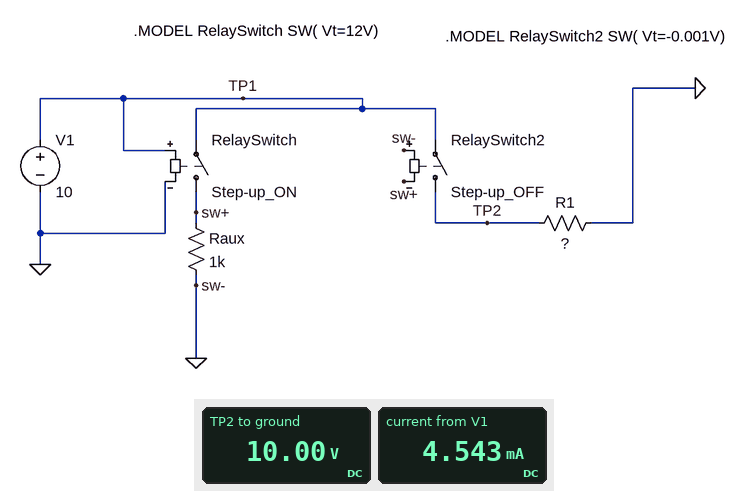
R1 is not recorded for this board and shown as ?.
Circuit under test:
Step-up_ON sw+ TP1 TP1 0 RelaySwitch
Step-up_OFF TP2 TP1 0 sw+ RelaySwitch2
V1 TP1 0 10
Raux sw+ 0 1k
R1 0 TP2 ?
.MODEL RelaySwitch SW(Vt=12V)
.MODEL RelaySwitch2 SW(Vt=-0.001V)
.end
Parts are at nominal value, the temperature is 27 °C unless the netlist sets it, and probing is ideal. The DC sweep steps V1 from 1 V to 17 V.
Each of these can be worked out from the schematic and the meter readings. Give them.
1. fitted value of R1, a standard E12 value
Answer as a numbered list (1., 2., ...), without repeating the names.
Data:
1. 2.2 kΩ
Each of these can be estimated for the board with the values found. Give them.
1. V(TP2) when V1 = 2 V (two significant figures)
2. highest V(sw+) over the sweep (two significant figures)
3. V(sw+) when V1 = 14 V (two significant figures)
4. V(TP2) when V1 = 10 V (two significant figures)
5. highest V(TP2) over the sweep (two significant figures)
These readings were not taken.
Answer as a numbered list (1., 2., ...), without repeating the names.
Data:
1. 2.0 V
2. 17 V
3. 14 V
4. 10 V
5. 12 V
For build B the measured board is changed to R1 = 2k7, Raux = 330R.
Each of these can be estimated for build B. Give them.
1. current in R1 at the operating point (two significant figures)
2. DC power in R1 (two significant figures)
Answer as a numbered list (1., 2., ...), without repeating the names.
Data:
1. 3.7 mA
2. 37 mW
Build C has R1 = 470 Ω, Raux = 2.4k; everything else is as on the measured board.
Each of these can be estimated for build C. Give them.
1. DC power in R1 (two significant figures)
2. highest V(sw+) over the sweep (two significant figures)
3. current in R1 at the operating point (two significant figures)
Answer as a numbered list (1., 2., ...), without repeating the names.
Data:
1. 210 mW
2. 17 V
3. 21 mA
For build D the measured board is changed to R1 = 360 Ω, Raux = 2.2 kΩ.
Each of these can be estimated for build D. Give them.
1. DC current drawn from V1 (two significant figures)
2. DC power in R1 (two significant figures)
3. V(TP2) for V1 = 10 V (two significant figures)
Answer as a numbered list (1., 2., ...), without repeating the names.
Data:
1. 28 mA
2. 280 mW
3. 10 V
